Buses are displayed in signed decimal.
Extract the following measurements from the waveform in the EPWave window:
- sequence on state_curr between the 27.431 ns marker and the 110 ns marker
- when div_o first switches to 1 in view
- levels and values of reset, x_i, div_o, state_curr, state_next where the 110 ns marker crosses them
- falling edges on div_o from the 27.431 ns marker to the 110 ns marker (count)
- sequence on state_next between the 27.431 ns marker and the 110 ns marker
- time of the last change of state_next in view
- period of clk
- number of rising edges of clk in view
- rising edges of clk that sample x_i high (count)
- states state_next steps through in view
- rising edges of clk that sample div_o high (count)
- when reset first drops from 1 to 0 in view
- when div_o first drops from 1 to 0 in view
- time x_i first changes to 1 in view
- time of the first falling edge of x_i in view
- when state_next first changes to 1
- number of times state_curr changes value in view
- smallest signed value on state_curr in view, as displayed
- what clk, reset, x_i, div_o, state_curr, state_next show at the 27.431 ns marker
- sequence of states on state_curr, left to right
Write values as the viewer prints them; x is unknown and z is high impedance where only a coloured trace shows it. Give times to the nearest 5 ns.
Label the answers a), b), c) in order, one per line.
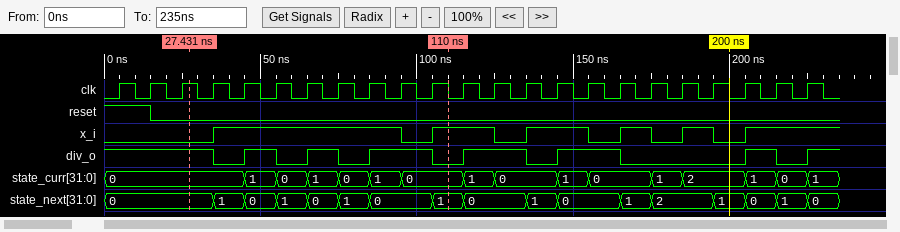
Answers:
a) 0, 1, 0, 1, 0, 1, 0
b) 45 ns
c) reset=0, x_i=1, div_o=0, state_curr=0, state_next=1
d) 4
e) 0, 1, 0, 1, 0, 1, 0, 1
f) 225 ns
g) 10 ns
h) 23
i) 14
j) 0, 1, 0, 1, 0, 1, 0, 1, 0, 1, 0, 1, 2, 1, 0, 1, 0
k) 13
l) 15 ns
m) 35 ns
n) 35 ns
o) 95 ns
p) 35 ns
q) 15
r) 0
s) clk=1, reset=0, x_i=0, div_o=1, state_curr=0, state_next=0
t) 0, 1, 0, 1, 0, 1, 0, 1, 0, 1, 0, 1, 2, 1, 0, 1
